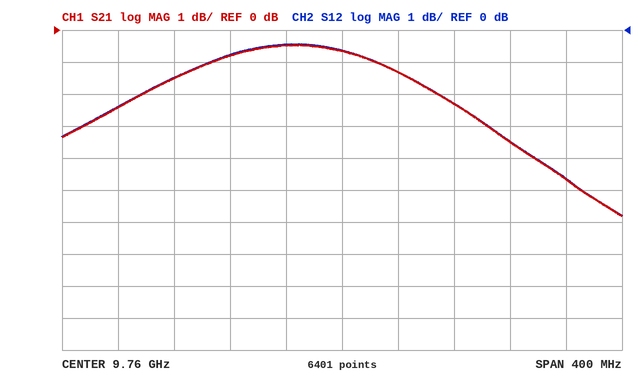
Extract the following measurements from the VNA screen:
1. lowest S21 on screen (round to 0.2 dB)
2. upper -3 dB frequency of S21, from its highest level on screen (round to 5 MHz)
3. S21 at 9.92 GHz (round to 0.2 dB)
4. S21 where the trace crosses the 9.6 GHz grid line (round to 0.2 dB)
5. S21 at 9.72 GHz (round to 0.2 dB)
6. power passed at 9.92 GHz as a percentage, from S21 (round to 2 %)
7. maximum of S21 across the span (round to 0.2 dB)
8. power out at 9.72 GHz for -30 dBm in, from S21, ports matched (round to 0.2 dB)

-5.8 dB
9.880 GHz
-4.6 dB
-2.4 dB
-0.4 dB
34 %
-0.4 dB
-30.4 dBm
